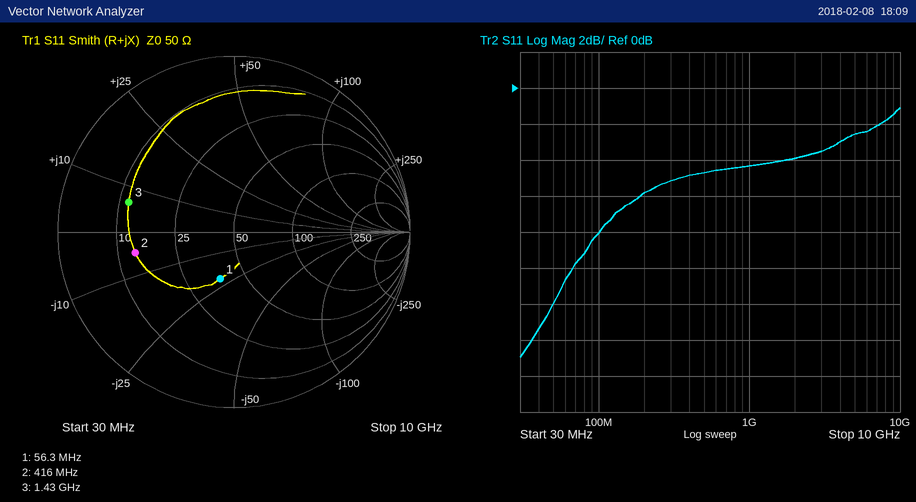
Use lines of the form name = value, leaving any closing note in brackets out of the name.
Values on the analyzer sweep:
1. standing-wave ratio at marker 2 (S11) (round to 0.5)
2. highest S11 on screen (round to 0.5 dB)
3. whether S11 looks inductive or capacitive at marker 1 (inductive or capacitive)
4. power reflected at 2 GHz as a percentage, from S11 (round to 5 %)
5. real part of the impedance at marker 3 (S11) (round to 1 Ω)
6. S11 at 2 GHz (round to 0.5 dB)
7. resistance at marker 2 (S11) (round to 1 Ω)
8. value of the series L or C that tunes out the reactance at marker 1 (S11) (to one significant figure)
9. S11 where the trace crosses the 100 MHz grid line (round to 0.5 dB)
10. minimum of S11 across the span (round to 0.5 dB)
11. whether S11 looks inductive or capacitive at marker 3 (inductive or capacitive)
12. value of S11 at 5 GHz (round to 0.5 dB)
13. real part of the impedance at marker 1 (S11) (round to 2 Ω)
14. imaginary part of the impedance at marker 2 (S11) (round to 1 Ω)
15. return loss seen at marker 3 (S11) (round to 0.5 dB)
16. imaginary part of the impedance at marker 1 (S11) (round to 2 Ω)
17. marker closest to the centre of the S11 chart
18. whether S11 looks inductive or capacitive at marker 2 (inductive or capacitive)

standing-wave ratio at marker 2 (S11) = 3.5
highest S11 on screen = -1.0 dB
whether S11 looks inductive or capacitive at marker 1 = capacitive
power reflected at 2 GHz as a percentage, from S11 = 40 %
real part of the impedance at marker 3 (S11) = 12 Ω
S11 at 2 GHz = -4.0 dB
resistance at marker 2 (S11) = 14 Ω
value of the series L or C that tunes out the reactance at marker 1 (S11) = 60 nH
S11 where the trace crosses the 100 MHz grid line = -8.0 dB
minimum of S11 across the span = -15.0 dB
whether S11 looks inductive or capacitive at marker 3 = inductive
value of S11 at 5 GHz = -2.5 dB
real part of the impedance at marker 1 (S11) = 38 Ω
imaginary part of the impedance at marker 2 (S11) = -5 Ω
return loss seen at marker 3 (S11) = 4.0 dB
imaginary part of the impedance at marker 1 (S11) = -22 Ω
marker closest to the centre of the S11 chart = marker 1
whether S11 looks inductive or capacitive at marker 2 = capacitive
